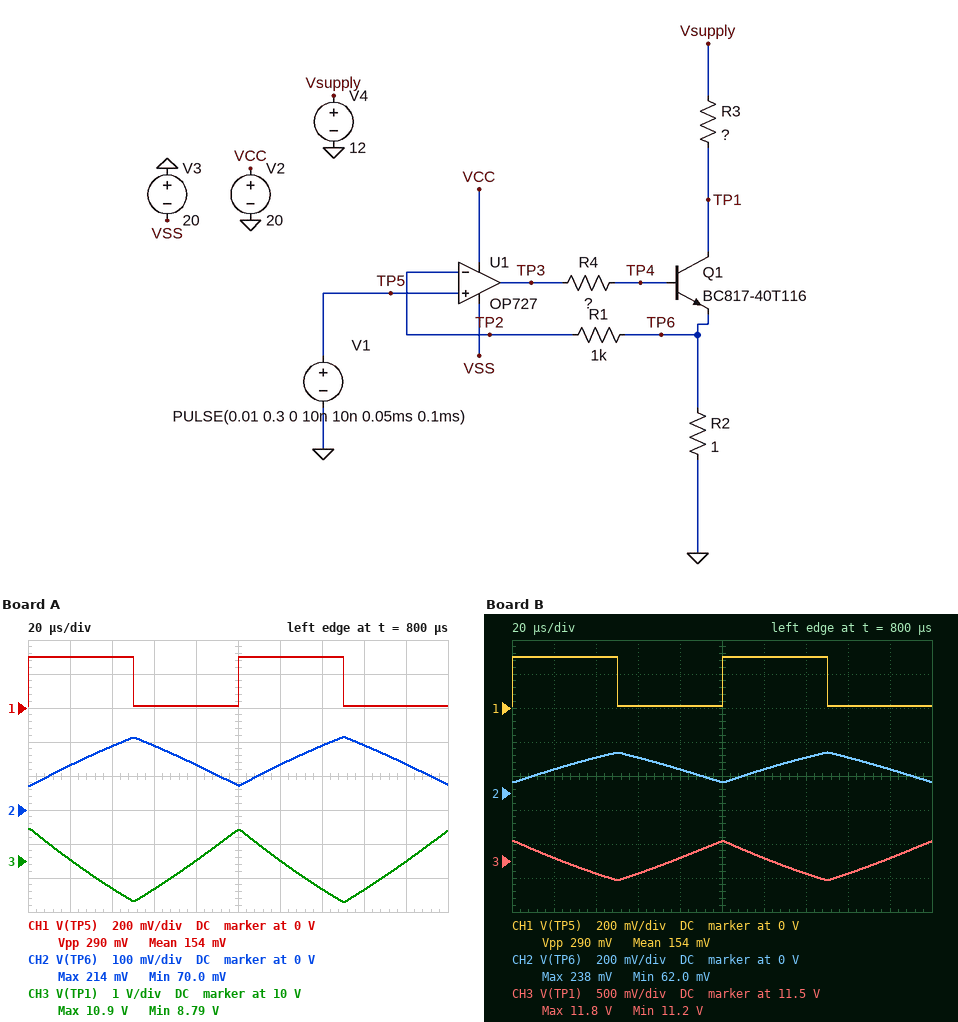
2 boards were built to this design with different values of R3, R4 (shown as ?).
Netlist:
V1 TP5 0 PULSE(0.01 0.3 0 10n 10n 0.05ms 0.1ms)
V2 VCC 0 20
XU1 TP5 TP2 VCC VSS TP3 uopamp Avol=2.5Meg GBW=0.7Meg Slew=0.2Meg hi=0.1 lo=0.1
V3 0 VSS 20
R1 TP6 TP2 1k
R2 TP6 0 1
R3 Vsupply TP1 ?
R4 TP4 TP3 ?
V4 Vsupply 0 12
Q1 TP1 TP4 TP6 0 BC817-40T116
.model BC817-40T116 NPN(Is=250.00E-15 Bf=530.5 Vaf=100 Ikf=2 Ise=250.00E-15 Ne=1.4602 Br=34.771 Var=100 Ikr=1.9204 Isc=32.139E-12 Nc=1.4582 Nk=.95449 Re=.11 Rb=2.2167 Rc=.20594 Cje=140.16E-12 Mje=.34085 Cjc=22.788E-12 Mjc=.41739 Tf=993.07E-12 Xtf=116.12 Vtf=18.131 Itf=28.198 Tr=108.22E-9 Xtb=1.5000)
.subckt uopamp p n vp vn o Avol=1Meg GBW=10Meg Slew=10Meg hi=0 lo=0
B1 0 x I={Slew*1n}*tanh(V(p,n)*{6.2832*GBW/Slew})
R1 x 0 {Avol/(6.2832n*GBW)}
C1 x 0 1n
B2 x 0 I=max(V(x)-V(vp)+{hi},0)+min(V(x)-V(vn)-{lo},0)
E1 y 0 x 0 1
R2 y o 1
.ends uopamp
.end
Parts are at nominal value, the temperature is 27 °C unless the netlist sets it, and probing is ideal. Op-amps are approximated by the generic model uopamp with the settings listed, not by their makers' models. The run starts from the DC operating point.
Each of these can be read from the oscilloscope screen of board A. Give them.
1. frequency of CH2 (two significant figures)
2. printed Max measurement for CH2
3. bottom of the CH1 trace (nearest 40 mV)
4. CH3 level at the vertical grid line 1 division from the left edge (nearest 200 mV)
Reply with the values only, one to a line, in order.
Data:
10 kHz
214 mV
0 V
10.0 V
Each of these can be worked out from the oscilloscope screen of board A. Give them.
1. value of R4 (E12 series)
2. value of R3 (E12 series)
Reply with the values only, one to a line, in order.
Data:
27 kΩ
15 Ω
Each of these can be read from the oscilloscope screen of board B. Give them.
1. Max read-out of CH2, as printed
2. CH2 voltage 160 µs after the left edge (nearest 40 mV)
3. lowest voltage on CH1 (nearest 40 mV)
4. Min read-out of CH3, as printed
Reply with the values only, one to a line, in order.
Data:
238 mV
200 mV
0 V
11.2 V
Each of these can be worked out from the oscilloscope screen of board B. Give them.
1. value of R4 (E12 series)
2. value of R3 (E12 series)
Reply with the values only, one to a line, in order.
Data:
22 kΩ
3.3 Ω
